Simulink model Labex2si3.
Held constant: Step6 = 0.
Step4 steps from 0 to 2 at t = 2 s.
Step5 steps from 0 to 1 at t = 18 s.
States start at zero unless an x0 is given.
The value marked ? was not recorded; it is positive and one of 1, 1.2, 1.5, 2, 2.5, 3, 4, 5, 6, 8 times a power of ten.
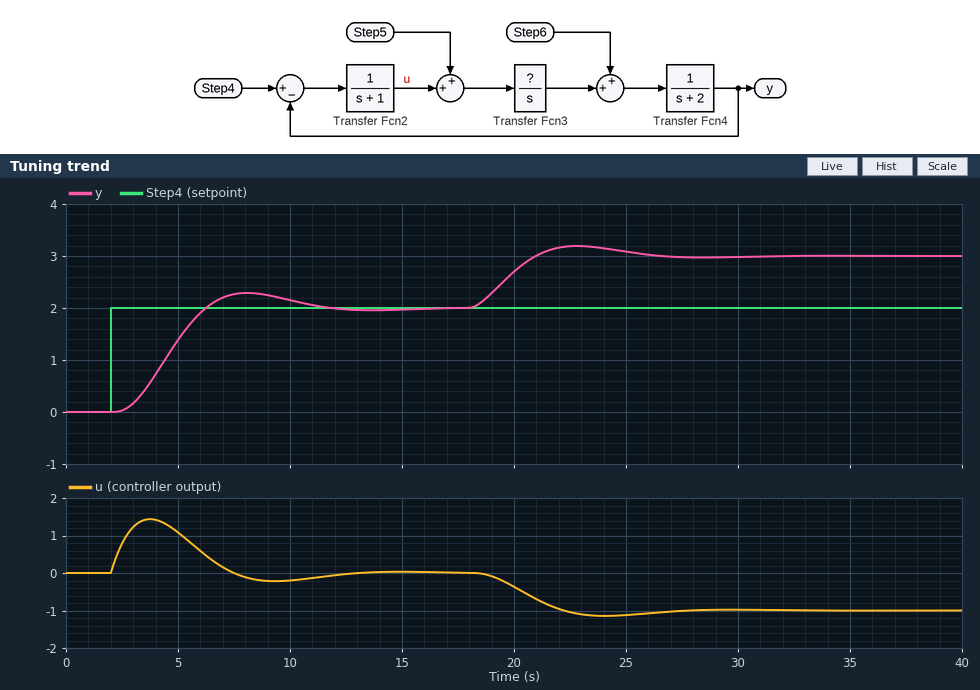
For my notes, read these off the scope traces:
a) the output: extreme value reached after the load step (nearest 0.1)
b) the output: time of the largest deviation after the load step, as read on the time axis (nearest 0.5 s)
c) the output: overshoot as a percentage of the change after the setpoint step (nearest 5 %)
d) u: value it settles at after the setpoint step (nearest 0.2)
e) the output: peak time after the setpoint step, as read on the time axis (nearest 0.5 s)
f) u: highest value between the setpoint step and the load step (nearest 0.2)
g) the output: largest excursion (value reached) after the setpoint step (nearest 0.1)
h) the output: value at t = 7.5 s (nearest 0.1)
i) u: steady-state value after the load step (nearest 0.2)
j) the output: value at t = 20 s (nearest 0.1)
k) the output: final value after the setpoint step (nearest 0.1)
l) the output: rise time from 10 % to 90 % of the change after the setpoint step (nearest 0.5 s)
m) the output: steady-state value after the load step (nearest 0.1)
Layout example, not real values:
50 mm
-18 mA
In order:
3.2
23.0 s
15 %
0.0
8.0 s
1.4
2.3
2.3
-1.0
2.7
2.0
2.5 s
3.0
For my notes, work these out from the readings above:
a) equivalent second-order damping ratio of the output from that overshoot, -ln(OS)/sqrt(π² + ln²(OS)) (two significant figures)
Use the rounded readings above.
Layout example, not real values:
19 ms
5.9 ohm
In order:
0.52
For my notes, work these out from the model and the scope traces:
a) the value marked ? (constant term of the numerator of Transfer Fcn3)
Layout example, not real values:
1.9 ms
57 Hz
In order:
1
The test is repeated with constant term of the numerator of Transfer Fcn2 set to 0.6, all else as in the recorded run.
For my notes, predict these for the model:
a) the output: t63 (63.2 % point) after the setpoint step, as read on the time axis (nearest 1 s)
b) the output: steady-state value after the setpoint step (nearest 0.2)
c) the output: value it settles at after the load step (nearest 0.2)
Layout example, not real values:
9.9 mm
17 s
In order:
6 s
2.0
3.6
